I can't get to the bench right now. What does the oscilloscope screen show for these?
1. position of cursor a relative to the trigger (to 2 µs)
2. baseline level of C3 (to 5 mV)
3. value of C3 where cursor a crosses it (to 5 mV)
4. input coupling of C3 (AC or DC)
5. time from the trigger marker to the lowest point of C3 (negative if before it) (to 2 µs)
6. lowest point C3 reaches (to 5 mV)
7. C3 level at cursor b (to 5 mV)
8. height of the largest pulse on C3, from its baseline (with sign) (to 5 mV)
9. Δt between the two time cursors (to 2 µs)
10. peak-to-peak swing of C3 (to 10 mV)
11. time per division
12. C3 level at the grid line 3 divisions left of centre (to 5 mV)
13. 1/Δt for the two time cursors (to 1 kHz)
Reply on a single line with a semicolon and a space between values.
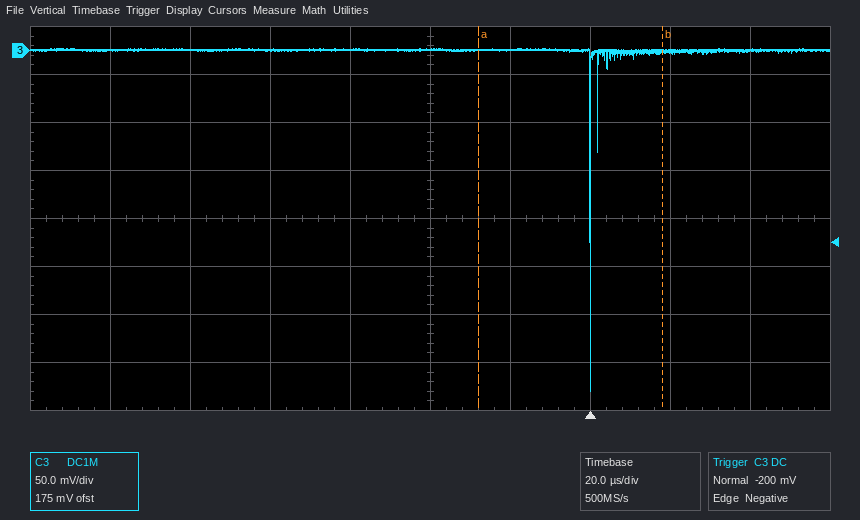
-28 µs; 0 mV; 0 mV; DC; 0 µs; -355 mV; 0 mV; -355 mV; 46 µs; 360 mV; 20 µs; 0 mV; 22 kHz
